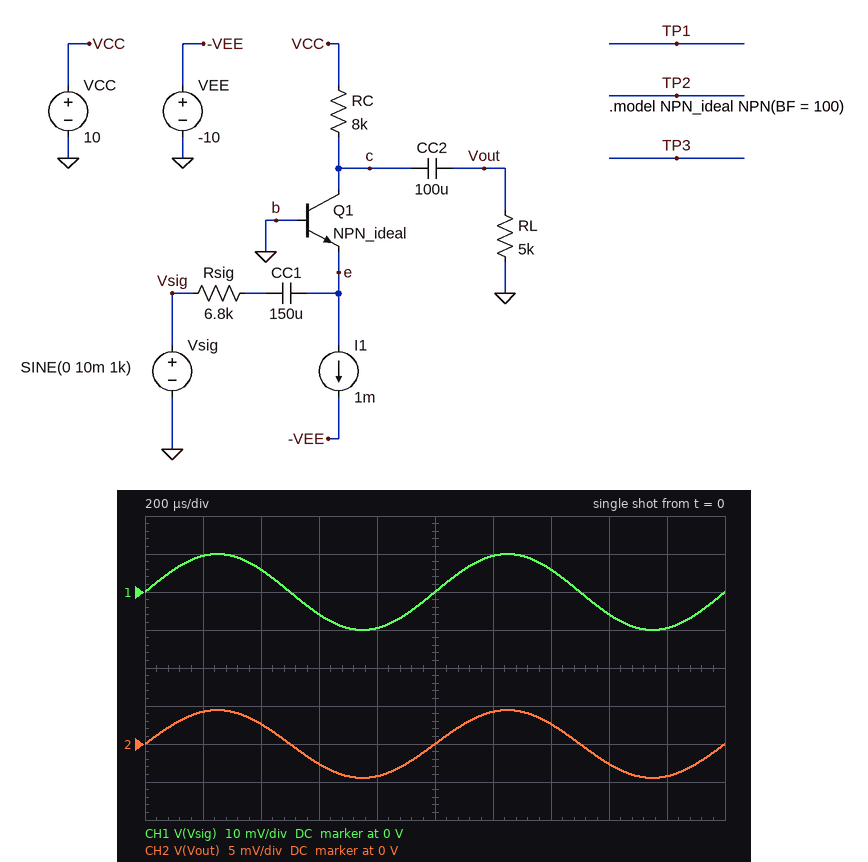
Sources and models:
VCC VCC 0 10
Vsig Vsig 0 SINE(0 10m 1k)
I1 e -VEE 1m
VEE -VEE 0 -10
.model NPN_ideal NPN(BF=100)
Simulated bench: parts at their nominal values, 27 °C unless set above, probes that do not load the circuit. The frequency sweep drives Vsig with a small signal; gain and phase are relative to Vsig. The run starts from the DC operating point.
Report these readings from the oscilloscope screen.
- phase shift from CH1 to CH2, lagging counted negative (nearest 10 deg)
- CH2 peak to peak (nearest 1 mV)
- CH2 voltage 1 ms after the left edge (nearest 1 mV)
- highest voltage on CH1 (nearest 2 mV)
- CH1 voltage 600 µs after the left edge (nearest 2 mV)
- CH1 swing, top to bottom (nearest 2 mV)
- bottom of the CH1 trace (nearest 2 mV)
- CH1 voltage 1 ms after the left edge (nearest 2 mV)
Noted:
0 deg
9 mV
0 V
10 mV
-6 mV
20 mV
-10 mV
0 V
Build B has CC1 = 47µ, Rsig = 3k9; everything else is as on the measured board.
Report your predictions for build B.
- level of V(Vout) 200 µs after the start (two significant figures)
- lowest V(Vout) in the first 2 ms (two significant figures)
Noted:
7.4 mV
-7.8 mV
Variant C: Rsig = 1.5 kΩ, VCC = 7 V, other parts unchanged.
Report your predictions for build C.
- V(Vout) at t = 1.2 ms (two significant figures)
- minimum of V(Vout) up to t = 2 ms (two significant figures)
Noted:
4.4 mV
-4.1 mV
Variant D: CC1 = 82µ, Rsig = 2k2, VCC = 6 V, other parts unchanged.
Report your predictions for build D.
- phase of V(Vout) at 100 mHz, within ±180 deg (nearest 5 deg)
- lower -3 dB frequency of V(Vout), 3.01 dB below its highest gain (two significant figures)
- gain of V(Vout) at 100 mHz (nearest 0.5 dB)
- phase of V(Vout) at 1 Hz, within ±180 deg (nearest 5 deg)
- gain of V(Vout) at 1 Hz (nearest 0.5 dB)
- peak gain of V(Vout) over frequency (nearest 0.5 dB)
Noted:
155 deg
960 mHz
-52.0 dB
60 deg
-25.5 dB
-23.0 dB
